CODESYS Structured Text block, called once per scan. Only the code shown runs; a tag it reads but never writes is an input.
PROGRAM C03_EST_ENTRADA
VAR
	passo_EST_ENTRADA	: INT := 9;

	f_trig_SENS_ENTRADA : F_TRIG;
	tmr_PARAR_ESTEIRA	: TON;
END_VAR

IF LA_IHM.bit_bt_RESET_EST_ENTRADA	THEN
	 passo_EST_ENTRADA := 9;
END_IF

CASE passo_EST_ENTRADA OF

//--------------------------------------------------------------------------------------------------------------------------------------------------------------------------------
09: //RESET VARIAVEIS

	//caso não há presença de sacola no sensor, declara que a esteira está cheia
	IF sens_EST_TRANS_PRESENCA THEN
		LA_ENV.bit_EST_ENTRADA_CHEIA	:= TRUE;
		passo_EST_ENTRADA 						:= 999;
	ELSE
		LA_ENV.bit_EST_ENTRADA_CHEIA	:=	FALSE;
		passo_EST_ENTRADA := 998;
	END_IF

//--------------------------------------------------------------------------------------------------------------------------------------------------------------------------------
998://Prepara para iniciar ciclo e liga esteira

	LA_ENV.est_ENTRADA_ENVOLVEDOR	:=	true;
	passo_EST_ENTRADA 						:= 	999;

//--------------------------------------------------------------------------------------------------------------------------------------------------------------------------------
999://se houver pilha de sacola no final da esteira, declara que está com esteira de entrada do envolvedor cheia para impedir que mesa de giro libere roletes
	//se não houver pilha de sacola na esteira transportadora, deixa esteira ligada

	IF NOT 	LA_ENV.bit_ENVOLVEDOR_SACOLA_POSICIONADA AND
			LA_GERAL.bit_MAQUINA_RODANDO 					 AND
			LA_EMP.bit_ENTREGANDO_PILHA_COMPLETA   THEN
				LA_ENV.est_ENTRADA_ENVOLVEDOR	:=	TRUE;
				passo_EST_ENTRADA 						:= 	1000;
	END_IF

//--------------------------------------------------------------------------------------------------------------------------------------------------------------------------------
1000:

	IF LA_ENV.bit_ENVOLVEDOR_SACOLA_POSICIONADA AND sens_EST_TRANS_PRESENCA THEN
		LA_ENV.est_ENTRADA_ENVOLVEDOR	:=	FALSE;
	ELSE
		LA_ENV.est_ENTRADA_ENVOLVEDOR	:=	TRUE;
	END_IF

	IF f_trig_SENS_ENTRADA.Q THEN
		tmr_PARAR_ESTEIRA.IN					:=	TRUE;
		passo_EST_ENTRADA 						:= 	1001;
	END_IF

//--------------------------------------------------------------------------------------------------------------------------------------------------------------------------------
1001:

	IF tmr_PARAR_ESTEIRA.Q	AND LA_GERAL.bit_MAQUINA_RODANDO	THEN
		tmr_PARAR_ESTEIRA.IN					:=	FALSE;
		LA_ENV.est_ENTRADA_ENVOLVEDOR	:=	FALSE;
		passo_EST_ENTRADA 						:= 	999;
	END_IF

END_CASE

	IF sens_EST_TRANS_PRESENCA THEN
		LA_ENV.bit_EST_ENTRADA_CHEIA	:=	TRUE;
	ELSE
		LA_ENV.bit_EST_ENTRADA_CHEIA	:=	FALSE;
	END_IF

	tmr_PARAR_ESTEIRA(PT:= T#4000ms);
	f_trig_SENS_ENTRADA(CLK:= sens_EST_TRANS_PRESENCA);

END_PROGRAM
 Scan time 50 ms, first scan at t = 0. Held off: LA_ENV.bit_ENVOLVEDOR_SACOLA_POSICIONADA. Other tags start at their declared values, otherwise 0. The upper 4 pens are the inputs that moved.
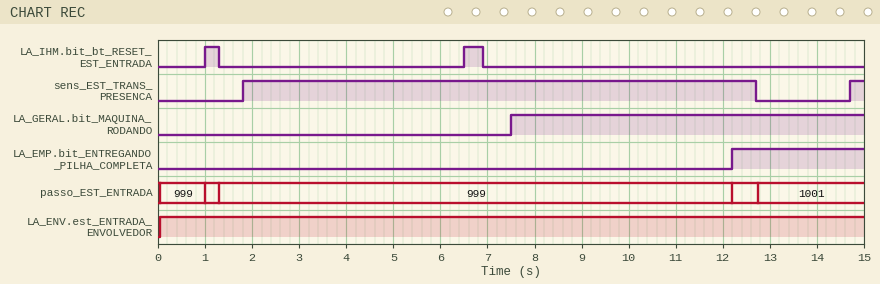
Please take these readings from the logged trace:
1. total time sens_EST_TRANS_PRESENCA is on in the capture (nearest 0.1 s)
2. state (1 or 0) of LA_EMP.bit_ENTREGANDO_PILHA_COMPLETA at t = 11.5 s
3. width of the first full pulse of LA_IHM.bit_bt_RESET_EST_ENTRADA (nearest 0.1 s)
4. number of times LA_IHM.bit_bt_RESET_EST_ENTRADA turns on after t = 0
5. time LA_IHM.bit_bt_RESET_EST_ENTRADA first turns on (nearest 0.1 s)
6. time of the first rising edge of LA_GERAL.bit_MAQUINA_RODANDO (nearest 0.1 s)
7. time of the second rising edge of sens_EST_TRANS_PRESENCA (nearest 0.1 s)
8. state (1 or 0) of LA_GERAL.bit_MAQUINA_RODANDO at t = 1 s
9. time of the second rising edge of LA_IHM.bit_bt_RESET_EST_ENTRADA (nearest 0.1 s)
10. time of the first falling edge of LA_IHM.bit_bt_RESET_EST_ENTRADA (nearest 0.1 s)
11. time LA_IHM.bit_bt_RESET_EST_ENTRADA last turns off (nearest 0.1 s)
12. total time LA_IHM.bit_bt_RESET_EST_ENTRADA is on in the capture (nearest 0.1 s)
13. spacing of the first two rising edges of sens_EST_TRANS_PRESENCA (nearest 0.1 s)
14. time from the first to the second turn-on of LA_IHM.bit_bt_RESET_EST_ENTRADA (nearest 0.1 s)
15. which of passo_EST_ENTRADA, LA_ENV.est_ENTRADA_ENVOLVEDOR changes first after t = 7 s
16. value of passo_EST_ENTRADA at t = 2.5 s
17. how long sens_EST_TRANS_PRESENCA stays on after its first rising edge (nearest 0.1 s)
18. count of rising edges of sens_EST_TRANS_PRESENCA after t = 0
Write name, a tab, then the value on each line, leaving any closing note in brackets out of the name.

total time sens_EST_TRANS_PRESENCA is on in the capture	11.2 s
state (1 or 0) of LA_EMP.bit_ENTREGANDO_PILHA_COMPLETA at t = 11.5 s	0
width of the first full pulse of LA_IHM.bit_bt_RESET_EST_ENTRADA	0.3 s
number of times LA_IHM.bit_bt_RESET_EST_ENTRADA turns on after t = 0	2
time LA_IHM.bit_bt_RESET_EST_ENTRADA first turns on	1.0 s
time of the first rising edge of LA_GERAL.bit_MAQUINA_RODANDO	7.5 s
time of the second rising edge of sens_EST_TRANS_PRESENCA	14.7 s
state (1 or 0) of LA_GERAL.bit_MAQUINA_RODANDO at t = 1 s	0
time of the second rising edge of LA_IHM.bit_bt_RESET_EST_ENTRADA	6.5 s
time of the first falling edge of LA_IHM.bit_bt_RESET_EST_ENTRADA	1.3 s
time LA_IHM.bit_bt_RESET_EST_ENTRADA last turns off	6.9 s
total time LA_IHM.bit_bt_RESET_EST_ENTRADA is on in the capture	0.7 s
spacing of the first two rising edges of sens_EST_TRANS_PRESENCA	12.9 s
time from the first to the second turn-on of LA_IHM.bit_bt_RESET_EST_ENTRADA	5.5 s
which of passo_EST_ENTRADA, LA_ENV.est_ENTRADA_ENVOLVEDOR changes first after t = 7 s	passo_EST_ENTRADA
value of passo_EST_ENTRADA at t = 2.5 s	999
how long sens_EST_TRANS_PRESENCA stays on after its first rising edge	10.9 s
count of rising edges of sens_EST_TRANS_PRESENCA after t = 0	2
